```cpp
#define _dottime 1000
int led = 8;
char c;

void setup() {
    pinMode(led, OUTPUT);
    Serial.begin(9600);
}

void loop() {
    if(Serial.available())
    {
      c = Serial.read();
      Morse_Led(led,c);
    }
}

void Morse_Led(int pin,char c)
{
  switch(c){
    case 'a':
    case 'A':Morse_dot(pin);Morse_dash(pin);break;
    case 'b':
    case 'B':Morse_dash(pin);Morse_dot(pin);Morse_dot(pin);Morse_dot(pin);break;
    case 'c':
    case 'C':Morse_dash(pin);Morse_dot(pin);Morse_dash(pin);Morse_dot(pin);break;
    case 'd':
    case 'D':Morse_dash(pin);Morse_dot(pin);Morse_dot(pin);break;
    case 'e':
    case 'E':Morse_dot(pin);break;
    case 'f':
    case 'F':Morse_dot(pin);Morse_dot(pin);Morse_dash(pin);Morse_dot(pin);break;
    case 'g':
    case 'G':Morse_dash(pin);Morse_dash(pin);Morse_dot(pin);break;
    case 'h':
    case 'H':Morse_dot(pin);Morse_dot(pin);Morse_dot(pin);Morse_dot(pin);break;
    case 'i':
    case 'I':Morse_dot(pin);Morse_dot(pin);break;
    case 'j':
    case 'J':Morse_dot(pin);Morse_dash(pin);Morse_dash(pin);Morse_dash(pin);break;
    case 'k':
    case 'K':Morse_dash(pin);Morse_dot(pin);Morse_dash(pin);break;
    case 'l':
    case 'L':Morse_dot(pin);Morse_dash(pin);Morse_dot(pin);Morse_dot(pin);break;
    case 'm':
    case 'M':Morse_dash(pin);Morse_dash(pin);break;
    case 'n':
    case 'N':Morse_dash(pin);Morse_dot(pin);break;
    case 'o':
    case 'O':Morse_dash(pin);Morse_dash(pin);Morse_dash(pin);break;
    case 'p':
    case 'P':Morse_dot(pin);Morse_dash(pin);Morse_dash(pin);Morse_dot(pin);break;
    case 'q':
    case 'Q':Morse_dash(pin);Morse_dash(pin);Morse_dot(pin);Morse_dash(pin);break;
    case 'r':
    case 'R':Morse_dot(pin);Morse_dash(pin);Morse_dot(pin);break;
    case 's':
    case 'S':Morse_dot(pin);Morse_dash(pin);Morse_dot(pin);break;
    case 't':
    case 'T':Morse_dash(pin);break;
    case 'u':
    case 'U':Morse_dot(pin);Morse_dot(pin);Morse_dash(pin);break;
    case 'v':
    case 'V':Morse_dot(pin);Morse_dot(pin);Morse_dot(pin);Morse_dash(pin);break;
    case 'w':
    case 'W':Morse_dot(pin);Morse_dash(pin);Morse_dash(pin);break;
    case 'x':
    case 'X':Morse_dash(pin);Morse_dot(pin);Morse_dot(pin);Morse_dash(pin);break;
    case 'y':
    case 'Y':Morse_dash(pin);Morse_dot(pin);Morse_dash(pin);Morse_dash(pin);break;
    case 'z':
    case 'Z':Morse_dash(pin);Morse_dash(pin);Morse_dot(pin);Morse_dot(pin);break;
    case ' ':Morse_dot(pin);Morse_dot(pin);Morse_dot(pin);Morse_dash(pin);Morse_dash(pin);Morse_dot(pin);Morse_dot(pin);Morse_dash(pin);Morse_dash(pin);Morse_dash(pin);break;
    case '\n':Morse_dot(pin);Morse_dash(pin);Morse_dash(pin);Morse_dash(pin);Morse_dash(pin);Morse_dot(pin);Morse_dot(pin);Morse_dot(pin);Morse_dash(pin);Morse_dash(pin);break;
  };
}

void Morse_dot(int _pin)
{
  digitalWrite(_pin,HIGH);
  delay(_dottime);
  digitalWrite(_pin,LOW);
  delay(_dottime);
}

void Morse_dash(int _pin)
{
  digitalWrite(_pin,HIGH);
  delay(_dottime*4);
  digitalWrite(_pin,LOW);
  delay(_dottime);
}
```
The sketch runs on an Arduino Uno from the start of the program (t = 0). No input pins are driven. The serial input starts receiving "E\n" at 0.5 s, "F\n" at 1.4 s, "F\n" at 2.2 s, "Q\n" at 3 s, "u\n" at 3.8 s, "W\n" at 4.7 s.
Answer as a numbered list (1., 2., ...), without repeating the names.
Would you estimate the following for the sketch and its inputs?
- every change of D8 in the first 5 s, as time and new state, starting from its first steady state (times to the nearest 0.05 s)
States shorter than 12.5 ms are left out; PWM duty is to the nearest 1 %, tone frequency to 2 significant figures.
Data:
1. 0 s low; 0.5 s high; 1.5 s low; 2.5 s high; 3.5 s low; 4.5 s high
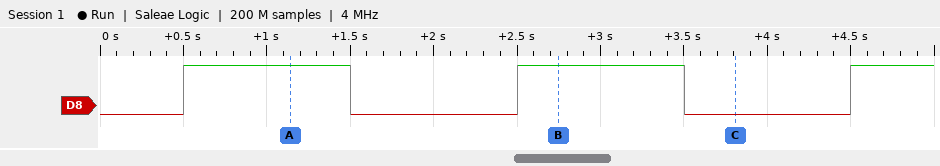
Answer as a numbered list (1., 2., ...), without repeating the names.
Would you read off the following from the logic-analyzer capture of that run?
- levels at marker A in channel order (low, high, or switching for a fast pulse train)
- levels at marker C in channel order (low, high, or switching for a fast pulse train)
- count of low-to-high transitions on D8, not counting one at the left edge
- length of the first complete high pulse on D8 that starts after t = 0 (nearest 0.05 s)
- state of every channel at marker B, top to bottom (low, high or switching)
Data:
1. D8 high
2. D8 low
3. 3
4. 1.00 s
5. D8 high
